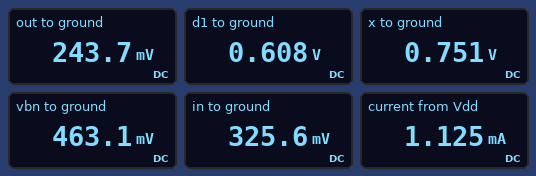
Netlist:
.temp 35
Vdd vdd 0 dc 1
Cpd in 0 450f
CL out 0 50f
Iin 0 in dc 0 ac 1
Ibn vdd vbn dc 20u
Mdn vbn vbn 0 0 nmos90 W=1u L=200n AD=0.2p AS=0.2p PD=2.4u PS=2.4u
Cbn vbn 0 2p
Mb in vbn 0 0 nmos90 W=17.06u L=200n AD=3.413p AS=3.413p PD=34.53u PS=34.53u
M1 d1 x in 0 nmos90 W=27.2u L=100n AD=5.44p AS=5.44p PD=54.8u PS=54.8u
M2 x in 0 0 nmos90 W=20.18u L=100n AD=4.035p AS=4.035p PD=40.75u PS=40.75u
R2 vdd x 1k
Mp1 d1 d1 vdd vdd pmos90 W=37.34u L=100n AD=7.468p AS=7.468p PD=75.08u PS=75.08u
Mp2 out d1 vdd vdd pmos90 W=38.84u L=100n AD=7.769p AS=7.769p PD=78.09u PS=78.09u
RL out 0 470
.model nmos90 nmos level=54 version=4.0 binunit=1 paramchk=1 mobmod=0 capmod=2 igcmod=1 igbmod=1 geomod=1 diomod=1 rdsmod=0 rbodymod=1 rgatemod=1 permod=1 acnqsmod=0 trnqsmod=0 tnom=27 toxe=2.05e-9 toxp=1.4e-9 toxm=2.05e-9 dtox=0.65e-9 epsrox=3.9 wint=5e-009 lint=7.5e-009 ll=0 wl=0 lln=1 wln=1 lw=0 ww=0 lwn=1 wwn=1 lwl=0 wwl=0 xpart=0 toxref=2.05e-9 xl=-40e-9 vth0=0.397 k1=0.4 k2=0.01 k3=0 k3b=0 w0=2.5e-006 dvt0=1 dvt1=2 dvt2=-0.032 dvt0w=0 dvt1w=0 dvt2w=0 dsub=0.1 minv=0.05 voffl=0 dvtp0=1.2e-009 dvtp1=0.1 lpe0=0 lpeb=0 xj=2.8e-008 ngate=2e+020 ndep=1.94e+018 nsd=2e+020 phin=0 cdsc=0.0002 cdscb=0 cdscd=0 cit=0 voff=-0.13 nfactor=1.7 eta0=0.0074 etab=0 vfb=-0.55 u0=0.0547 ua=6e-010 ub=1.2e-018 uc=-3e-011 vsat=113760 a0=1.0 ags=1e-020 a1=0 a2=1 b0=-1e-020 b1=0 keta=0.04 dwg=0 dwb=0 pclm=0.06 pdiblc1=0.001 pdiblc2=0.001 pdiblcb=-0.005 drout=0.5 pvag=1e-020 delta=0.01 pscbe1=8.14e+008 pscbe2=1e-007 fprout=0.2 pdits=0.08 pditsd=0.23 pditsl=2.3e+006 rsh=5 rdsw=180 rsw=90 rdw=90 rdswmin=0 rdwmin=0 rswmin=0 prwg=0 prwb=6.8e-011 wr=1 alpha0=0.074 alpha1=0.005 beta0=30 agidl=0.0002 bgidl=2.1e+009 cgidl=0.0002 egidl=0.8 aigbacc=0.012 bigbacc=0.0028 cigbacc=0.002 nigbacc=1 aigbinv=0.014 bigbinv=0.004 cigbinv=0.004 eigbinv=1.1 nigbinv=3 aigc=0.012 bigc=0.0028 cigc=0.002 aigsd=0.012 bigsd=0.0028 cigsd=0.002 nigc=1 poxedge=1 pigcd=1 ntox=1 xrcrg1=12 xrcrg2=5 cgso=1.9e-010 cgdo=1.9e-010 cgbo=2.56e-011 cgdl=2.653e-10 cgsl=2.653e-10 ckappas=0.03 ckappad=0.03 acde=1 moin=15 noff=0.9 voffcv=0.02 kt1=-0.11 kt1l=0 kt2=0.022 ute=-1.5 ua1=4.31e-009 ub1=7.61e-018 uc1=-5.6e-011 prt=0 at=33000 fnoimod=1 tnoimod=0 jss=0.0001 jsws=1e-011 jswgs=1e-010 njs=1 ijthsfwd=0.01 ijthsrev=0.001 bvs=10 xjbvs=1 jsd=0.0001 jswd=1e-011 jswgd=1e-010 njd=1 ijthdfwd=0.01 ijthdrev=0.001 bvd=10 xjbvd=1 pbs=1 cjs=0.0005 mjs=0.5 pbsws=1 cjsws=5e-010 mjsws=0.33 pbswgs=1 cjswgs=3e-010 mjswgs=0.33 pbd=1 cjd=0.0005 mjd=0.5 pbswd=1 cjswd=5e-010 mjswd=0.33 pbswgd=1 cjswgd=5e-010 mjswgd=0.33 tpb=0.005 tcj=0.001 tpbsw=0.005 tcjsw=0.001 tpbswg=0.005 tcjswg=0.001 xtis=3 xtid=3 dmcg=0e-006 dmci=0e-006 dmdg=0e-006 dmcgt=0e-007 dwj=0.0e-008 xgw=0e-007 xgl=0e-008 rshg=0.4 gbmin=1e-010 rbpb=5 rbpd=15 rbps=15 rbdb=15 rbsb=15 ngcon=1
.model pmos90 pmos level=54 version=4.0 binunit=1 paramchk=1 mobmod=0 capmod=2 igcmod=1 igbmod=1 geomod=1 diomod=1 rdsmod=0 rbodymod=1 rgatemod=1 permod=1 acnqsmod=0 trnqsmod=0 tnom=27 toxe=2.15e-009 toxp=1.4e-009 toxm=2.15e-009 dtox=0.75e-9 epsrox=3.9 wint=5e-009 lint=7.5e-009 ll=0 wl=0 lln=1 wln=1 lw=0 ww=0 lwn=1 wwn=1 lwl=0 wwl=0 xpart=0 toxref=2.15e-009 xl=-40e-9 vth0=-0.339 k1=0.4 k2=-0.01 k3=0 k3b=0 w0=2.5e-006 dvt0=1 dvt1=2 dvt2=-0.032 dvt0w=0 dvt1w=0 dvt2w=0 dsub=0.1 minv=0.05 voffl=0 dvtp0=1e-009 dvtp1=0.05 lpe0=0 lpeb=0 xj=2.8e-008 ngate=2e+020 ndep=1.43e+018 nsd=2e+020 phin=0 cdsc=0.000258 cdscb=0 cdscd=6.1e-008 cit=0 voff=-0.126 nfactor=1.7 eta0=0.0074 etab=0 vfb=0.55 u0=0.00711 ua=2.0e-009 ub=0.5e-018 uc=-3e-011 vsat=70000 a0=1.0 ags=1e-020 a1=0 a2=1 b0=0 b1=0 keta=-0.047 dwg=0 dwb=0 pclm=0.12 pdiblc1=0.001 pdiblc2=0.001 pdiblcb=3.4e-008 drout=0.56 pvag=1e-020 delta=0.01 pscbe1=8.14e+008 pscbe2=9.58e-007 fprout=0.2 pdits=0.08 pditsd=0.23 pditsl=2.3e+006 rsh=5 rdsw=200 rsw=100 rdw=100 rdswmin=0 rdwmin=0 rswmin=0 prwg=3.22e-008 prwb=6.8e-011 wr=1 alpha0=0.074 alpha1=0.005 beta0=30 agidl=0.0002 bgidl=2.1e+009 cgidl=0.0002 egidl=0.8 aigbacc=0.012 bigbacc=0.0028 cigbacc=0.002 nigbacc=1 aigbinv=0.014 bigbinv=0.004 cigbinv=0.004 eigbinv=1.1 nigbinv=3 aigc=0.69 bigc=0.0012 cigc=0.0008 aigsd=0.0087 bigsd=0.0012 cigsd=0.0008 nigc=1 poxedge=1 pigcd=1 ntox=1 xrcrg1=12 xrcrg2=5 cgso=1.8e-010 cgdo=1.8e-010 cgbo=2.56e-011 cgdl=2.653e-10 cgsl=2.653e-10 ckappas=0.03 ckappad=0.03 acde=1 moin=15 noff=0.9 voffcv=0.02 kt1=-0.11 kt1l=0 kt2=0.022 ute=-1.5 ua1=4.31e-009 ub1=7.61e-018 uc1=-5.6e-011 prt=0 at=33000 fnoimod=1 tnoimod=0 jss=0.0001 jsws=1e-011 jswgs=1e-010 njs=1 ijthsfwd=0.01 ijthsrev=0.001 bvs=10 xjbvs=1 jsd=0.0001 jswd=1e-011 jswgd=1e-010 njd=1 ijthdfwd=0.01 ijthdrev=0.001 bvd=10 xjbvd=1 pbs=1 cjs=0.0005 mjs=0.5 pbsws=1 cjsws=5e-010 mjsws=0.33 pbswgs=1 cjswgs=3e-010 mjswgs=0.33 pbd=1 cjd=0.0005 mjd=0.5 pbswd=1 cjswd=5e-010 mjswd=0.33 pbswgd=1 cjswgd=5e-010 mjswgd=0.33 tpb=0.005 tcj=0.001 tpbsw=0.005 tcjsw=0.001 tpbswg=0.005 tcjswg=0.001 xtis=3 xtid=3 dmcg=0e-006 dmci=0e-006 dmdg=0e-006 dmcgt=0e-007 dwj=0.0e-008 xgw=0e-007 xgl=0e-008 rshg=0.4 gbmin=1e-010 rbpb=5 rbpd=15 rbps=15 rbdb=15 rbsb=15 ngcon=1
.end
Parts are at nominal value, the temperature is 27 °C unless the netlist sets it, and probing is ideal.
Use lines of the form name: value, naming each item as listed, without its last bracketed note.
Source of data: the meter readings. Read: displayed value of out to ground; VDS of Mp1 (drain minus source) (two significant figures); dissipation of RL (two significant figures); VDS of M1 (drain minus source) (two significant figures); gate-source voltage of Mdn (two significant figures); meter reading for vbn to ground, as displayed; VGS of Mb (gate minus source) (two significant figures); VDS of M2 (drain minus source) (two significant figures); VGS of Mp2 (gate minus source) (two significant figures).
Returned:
displayed value of out to ground: 243.7 mV
VDS of Mp1 (drain minus source): -390 mV
dissipation of RL: 130 µW
VDS of M1 (drain minus source): 280 mV
gate-source voltage of Mdn: 460 mV
meter reading for vbn to ground, as displayed: 463.1 mV
VGS of Mb (gate minus source): 460 mV
VDS of M2 (drain minus source): 750 mV
VGS of Mp2 (gate minus source): -390 mV
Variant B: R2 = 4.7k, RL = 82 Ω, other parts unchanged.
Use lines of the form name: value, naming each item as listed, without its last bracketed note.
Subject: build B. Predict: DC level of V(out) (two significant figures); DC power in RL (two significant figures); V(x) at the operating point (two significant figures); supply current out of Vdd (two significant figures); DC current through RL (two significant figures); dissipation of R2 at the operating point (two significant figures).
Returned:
DC level of V(out): 51 mV
DC power in RL: 31 µW
V(x) at the operating point: 670 mV
supply current out of Vdd: 1.0 mA
DC current through RL: 620 µA
dissipation of R2 at the operating point: 23 µW
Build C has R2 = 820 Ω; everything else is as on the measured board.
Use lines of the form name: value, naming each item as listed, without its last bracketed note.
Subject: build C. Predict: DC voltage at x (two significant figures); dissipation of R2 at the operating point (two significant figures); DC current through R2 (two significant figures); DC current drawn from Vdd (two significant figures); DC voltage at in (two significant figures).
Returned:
DC voltage at x: 760 mV
dissipation of R2 at the operating point: 69 µW
DC current through R2: 290 µA
DC current drawn from Vdd: 1.2 mA
DC voltage at in: 330 mV
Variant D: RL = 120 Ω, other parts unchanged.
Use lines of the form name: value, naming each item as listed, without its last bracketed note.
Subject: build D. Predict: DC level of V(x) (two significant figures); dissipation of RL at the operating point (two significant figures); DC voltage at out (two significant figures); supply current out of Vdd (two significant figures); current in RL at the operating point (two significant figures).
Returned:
DC level of V(x): 750 mV
dissipation of RL at the operating point: 45 µW
DC voltage at out: 73 mV
supply current out of Vdd: 1.2 mA
current in RL at the operating point: 610 µA
